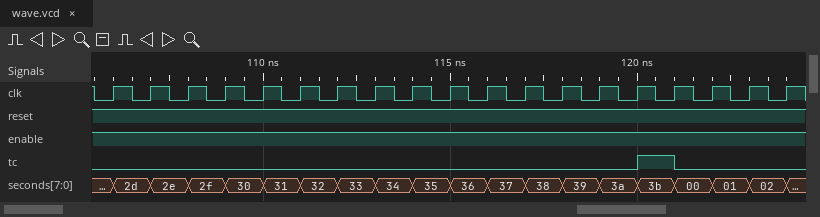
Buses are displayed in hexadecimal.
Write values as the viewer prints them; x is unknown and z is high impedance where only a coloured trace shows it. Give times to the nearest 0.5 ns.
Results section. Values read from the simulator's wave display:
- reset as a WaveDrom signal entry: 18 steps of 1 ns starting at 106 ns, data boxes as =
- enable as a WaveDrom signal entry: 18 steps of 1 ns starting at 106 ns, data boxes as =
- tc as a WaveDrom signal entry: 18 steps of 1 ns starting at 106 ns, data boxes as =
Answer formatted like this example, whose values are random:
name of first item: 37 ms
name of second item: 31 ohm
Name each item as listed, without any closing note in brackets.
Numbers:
reset as a WaveDrom signal entry: 18 steps of 1 ns starting at 106 ns, data boxes as =: {name: 'reset', wave: '1.................'}
enable as a WaveDrom signal entry: 18 steps of 1 ns starting at 106 ns, data boxes as =: {name: 'enable', wave: '1.................'}
tc as a WaveDrom signal entry: 18 steps of 1 ns starting at 106 ns, data boxes as =: {name: 'tc', wave: '0.............10..'}
